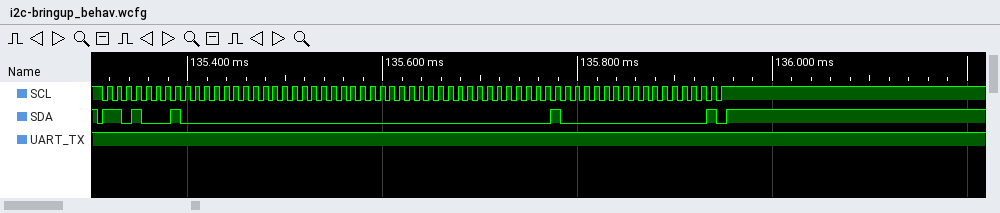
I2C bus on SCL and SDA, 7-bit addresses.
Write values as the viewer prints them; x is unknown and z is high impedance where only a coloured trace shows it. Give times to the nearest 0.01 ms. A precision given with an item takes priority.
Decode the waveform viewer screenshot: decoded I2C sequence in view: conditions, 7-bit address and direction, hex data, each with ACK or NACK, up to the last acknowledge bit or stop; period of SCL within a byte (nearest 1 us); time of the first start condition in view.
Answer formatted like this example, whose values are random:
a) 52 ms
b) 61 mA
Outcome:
a) start, address 68 read ACK, 00 ACK, 00 ACK, 00 ACK, 00 ACK, 40 ACK, 00 NACK, stop
b) 10 us
c) 135.31 ms
